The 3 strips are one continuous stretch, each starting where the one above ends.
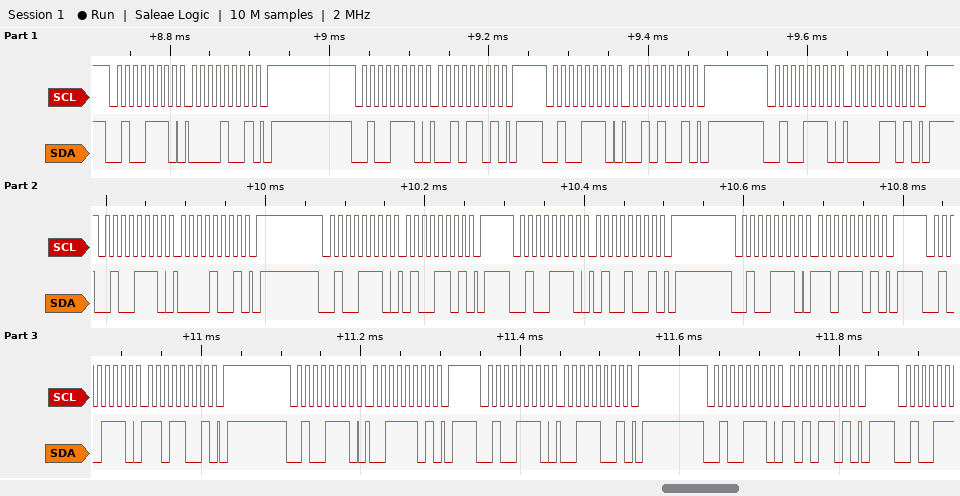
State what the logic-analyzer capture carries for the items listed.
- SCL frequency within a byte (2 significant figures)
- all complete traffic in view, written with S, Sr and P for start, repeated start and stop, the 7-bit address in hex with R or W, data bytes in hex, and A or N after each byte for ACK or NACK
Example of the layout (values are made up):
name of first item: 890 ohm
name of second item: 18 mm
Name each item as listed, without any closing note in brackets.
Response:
SCL frequency within a byte: 100 kHz
all complete traffic in view, written with S, Sr and P for start, repeated start and stop, the 7-bit address in hex with R or W, data bytes in hex, and A or N after each byte for ACK or NACK: S 27W A 09 A P S 27W A 2D A P S 27W A 29 A P S 27W A 0D A P S 27W A 09 A P S 27W A 4D A P S 27W A 49 A P S 27W A DD A P S 27W A D9 A P S 27W A 3D A P S 27W A 39 A P S 27W A AD A P
